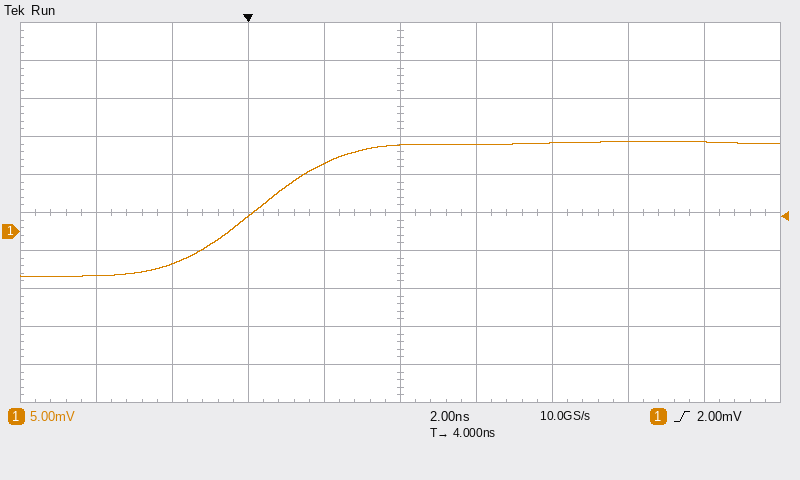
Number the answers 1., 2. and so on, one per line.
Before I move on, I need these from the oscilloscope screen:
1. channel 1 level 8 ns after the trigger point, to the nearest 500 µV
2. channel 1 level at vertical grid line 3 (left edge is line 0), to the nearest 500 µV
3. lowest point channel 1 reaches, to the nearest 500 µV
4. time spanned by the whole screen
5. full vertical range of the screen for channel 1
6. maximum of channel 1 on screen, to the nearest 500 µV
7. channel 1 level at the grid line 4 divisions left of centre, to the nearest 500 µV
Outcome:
1. 11.5 mV
2. 2.0 mV
3. -6.0 mV
4. 20 ns
5. 50 mV
6. 12.0 mV
7. -6.0 mV
